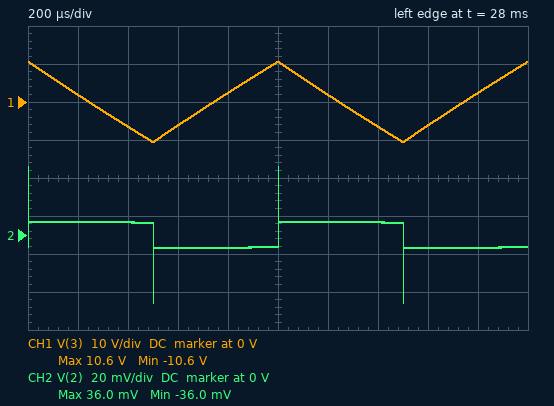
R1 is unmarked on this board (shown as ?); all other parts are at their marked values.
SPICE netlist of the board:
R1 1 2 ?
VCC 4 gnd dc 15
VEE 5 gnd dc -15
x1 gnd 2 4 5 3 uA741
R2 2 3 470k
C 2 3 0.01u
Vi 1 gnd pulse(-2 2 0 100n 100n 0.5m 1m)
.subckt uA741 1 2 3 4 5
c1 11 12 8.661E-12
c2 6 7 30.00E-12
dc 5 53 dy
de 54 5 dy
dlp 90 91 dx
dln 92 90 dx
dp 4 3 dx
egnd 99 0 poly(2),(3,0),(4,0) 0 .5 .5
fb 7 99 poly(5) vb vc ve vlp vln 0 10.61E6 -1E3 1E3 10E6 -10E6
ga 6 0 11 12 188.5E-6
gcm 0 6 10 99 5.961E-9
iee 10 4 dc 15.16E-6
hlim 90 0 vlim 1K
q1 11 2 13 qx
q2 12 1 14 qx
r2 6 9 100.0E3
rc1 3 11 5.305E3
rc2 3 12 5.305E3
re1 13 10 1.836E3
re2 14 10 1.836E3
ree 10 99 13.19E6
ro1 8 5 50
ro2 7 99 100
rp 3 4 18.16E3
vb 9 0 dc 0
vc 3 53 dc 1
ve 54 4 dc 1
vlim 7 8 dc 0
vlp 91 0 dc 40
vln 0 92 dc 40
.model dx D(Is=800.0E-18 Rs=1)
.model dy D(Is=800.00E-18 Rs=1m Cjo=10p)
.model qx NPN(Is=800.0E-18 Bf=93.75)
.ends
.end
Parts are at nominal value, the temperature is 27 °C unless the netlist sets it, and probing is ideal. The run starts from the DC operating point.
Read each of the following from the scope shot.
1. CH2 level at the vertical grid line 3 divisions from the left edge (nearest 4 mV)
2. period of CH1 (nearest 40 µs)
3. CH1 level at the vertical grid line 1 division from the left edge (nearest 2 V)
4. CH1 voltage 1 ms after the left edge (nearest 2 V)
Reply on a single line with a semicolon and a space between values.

-8 mV; 1.00 ms; 2 V; 10 V
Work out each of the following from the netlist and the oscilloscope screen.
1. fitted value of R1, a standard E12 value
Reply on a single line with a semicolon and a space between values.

4.7 kΩ
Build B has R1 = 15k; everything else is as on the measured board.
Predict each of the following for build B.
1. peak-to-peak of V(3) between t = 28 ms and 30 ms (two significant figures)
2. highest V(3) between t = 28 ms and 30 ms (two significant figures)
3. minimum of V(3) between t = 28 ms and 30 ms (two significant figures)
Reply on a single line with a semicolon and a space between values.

6.7 V; 3.4 V; -3.3 V
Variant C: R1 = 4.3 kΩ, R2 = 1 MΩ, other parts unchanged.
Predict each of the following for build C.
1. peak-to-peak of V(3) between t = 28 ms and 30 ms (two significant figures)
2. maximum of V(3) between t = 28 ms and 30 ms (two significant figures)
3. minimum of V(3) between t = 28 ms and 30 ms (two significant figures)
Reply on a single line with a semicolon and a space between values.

23 V; 12 V; -11 V
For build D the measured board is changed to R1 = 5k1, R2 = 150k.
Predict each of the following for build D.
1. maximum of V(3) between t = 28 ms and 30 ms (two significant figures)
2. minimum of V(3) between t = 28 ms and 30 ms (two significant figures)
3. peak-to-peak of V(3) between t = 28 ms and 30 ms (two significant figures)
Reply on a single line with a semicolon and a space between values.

9.7 V; -9.7 V; 19 V
